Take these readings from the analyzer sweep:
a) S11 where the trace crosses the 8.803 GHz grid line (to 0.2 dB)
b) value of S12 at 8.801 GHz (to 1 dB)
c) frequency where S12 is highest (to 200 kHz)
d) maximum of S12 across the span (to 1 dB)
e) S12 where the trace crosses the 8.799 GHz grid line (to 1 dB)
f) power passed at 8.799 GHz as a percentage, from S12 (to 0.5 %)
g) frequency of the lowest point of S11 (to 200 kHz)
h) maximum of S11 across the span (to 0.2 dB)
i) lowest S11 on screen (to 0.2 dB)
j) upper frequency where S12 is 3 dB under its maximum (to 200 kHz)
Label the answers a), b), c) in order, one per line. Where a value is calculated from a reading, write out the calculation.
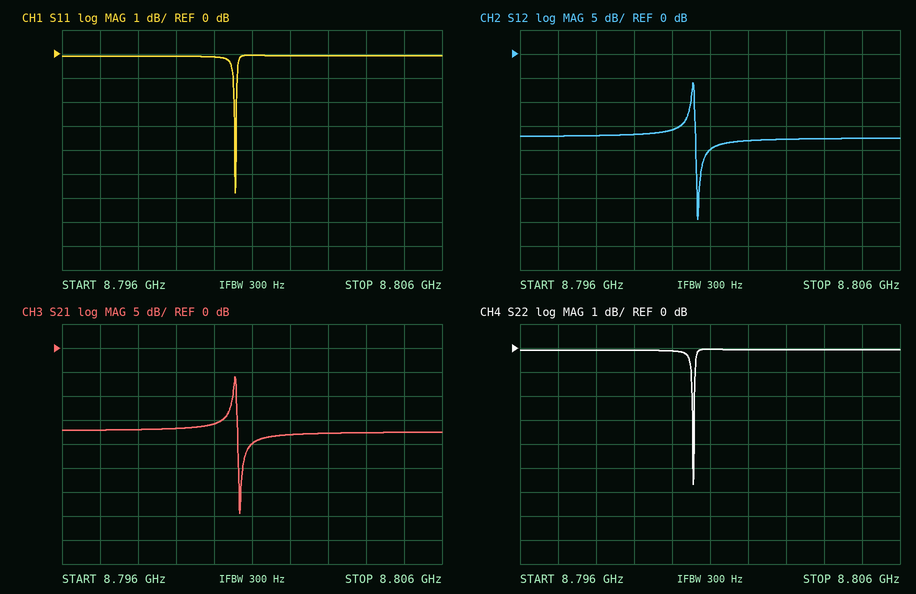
a) 0.0 dB
b) -20 dB
c) 8.8006 GHz
d) -6 dB
e) -17 dB
f) 10^(-17/10) ≈ 2.0 %
g) 8.8006 GHz
h) 0.0 dB
i) -5.8 dB
j) 8.8006 GHz
